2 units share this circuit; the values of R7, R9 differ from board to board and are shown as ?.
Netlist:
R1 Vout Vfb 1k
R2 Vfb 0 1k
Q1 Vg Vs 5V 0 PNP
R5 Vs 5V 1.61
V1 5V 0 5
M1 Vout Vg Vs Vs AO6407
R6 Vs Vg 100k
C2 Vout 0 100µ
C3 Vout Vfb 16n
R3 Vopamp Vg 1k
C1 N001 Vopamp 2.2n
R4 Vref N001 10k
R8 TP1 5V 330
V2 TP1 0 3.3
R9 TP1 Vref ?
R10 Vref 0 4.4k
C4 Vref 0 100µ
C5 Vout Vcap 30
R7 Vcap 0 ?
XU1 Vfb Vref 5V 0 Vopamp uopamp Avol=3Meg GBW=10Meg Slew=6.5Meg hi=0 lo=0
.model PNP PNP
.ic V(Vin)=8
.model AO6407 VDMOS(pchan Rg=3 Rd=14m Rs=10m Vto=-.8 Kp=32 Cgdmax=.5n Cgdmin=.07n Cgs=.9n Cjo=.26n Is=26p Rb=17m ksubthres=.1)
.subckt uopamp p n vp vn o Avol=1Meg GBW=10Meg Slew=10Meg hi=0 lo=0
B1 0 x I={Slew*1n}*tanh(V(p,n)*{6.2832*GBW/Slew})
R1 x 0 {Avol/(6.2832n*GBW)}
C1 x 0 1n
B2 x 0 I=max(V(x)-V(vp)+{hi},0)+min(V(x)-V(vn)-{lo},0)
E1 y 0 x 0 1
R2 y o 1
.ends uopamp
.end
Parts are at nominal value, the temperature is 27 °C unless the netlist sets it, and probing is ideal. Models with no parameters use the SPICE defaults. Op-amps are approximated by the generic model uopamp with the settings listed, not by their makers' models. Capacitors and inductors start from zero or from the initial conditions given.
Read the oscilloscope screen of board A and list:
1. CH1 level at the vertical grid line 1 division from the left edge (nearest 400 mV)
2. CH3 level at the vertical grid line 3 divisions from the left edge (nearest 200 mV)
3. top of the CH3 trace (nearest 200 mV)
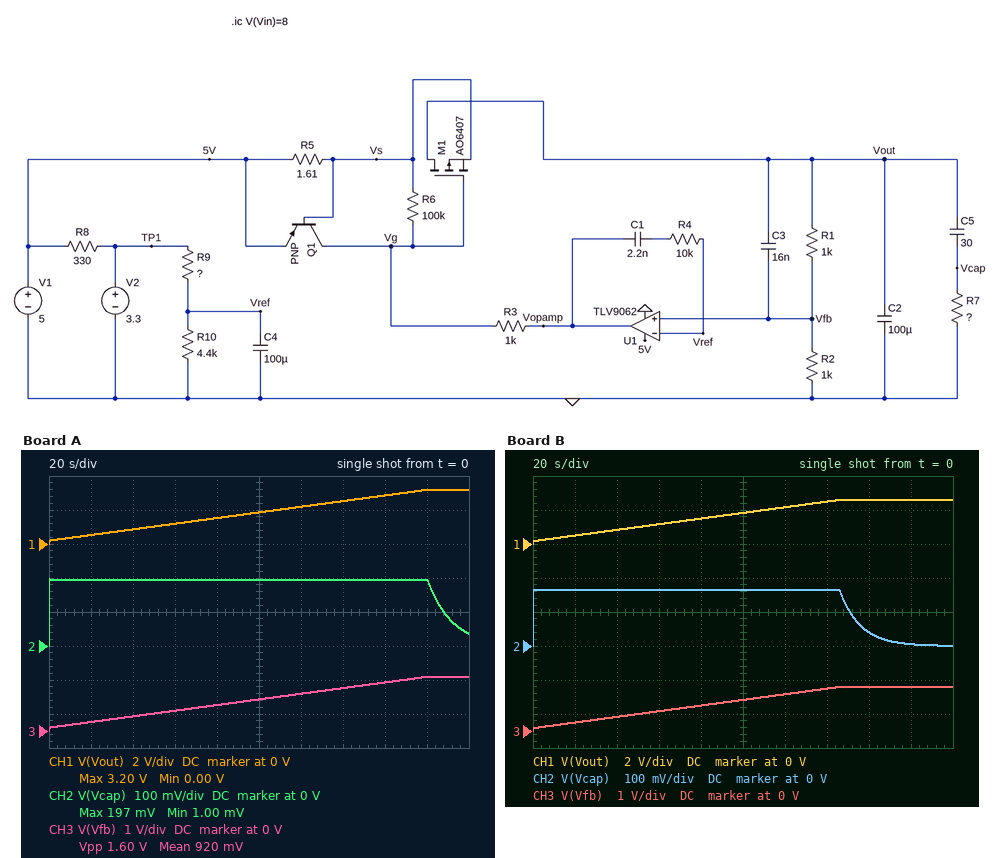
400 mV
600 mV
1.6 V
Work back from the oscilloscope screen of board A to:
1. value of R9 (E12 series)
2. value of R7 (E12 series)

4.7 kΩ
0.39 Ω
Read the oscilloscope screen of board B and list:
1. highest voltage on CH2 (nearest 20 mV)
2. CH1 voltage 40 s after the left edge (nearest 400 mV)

160 mV
800 mV
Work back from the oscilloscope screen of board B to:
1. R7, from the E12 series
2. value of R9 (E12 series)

0.33 Ω
6.8 kΩ
